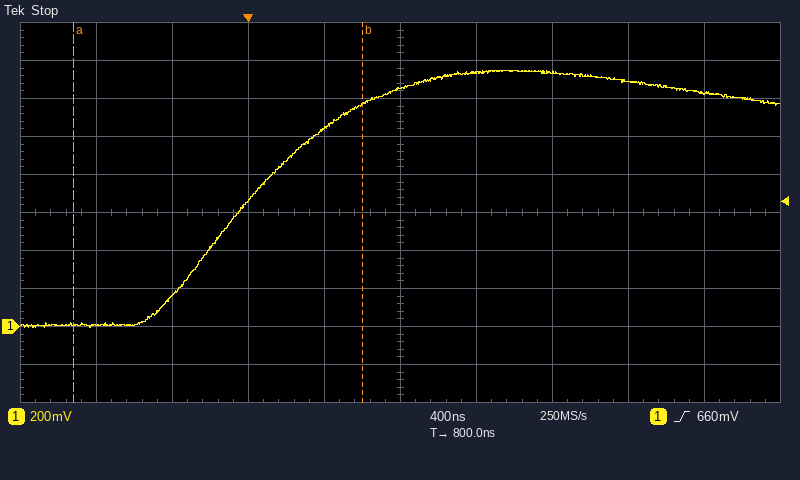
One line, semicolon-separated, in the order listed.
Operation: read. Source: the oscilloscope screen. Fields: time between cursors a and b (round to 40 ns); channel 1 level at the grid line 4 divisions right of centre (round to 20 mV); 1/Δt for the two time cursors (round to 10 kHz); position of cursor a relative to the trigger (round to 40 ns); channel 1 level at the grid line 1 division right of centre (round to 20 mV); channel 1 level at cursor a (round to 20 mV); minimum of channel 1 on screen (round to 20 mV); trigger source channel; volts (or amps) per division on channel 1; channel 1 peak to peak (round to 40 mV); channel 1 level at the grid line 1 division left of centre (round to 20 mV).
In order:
1.52 µs; 1.22 V; 660 kHz; -920 ns; 1.34 V; 20 mV; 0 mV; channel 1; 200 mV; 1.36 V; 1.04 V
